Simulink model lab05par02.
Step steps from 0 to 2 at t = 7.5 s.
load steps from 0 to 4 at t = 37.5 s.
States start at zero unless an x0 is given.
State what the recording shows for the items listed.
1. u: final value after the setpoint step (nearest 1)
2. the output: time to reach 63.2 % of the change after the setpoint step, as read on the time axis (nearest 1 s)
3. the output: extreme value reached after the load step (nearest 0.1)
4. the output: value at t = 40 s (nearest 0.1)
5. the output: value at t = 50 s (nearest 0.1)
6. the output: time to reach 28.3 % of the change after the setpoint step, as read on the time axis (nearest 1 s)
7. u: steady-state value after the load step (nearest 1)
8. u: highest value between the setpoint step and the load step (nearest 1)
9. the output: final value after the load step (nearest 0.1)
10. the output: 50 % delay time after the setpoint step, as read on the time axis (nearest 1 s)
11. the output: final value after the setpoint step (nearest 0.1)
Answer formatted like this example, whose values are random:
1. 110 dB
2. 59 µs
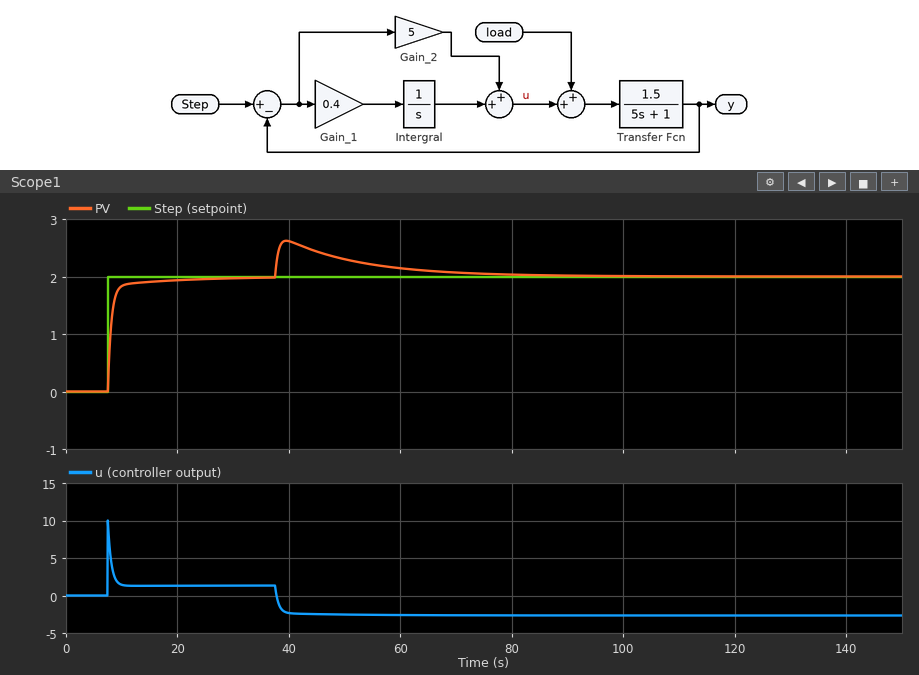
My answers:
1. 1
2. 8 s
3. 2.6
4. 2.6
5. 2.3
6. 8 s
7. -3
8. 10
9. 2.0
10. 8 s
11. 2.0
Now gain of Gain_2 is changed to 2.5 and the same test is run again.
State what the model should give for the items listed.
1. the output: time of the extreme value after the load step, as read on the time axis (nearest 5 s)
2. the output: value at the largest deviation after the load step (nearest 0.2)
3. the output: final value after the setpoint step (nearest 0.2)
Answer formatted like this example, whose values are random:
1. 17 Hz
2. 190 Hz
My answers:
1. 40 s
2. 3.0
3. 2.0
